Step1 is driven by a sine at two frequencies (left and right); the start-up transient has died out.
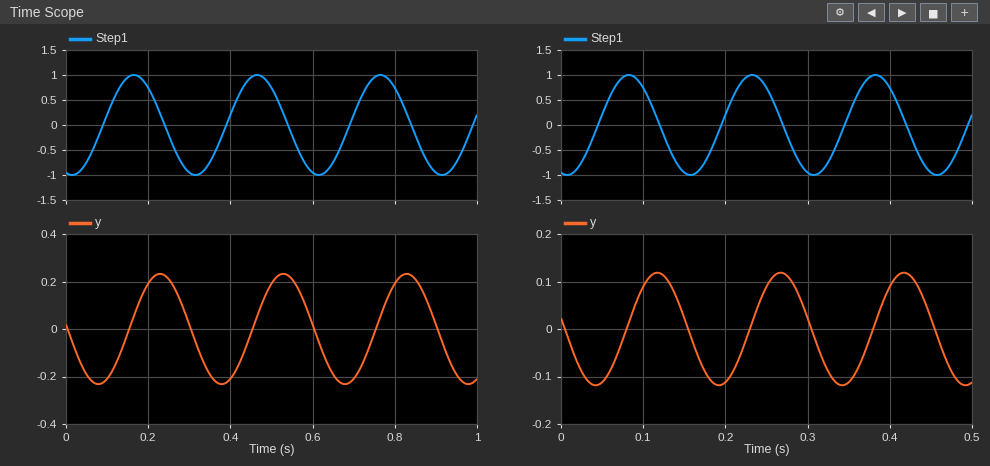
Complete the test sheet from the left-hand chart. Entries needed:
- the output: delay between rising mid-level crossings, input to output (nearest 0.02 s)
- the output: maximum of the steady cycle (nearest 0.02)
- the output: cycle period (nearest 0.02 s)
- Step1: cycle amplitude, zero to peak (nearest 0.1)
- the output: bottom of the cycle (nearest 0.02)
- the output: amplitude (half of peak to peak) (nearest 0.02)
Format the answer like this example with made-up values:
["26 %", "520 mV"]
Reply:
["0.06 s", "0.24", "0.30 s", "1.0", "-0.24", "0.24"]
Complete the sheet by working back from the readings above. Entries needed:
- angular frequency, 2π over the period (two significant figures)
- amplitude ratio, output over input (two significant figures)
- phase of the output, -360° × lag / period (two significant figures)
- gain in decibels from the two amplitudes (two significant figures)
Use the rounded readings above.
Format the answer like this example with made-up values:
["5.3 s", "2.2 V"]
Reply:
["21 rad/s", "0.24", "-72°", "-12 dB"]
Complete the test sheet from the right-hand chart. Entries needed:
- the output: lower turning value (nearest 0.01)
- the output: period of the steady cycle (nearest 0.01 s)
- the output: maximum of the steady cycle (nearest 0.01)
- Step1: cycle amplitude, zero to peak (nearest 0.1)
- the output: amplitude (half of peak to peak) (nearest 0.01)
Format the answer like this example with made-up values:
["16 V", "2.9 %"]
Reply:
["-0.12", "0.15 s", "0.12", "1.0", "0.12"]
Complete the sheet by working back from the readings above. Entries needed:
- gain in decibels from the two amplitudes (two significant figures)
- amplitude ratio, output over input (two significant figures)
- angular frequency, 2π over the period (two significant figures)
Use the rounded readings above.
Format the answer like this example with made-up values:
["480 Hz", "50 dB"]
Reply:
["-18 dB", "0.12", "42 rad/s"]
